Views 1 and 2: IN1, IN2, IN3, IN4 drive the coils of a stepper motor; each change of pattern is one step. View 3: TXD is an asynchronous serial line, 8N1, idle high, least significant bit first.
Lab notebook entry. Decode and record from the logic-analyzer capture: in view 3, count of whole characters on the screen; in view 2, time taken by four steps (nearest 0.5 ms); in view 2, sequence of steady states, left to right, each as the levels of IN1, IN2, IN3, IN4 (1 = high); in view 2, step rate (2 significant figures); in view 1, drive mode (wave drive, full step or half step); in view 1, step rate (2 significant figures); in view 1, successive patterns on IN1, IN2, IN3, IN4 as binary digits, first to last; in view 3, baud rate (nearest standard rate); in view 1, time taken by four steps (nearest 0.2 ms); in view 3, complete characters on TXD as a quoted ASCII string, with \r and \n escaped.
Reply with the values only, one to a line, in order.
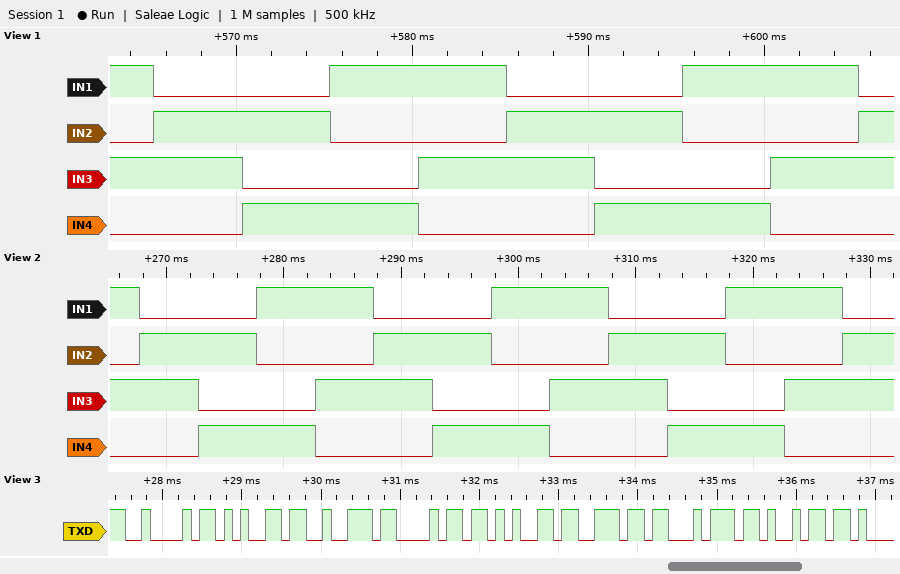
8
20.0 ms
1010 0110 0101 1001 1010 0110 0101 1001 1010 0110 0101 1001 1010 0110
200 steps/s
full step
200 steps/s
1010 0110 0101 1001 1010 0110 0101 1001 1010 0110
9600 baud
20.0 ms
"Berhenti"
